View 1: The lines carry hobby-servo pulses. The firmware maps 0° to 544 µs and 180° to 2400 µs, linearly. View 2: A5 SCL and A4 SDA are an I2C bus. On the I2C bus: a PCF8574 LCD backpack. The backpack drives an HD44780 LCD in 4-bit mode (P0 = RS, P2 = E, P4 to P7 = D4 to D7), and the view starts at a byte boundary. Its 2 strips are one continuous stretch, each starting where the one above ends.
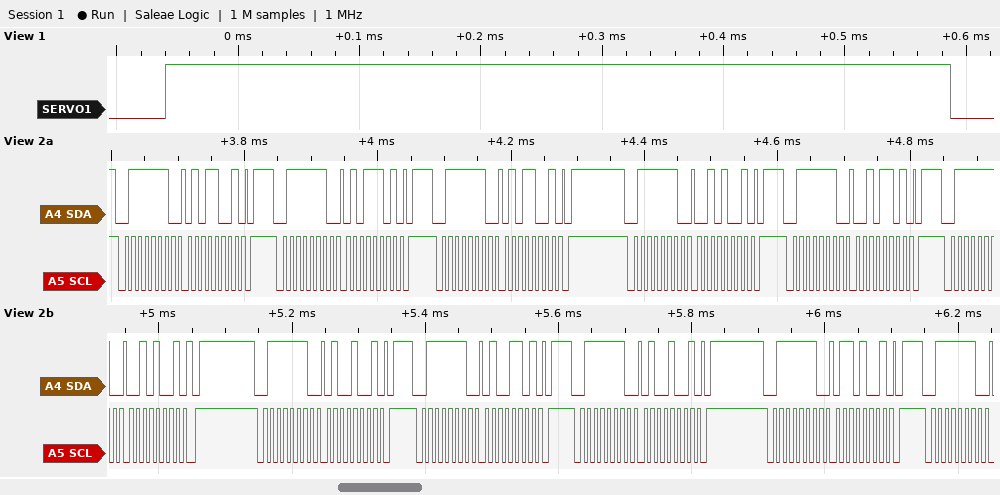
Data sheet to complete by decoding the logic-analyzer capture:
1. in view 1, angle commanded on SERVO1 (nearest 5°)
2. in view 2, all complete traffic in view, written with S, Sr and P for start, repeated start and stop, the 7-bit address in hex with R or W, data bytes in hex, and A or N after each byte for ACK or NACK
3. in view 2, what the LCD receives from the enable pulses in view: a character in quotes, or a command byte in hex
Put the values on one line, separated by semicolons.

10°; S 3FW A 59 A P S 3FW A 5D A P S 3FW A 59 A P S 3FW A 29 A P S 3FW A 2D A P S 3FW A 29 A P S 3FW A 49 A P S 3FW A 4D A P S 3FW A 49 A P S 3FW A 69 A P S 3FW A; 'R'
